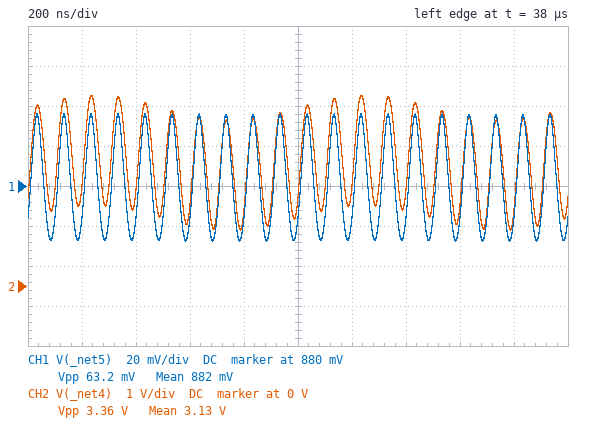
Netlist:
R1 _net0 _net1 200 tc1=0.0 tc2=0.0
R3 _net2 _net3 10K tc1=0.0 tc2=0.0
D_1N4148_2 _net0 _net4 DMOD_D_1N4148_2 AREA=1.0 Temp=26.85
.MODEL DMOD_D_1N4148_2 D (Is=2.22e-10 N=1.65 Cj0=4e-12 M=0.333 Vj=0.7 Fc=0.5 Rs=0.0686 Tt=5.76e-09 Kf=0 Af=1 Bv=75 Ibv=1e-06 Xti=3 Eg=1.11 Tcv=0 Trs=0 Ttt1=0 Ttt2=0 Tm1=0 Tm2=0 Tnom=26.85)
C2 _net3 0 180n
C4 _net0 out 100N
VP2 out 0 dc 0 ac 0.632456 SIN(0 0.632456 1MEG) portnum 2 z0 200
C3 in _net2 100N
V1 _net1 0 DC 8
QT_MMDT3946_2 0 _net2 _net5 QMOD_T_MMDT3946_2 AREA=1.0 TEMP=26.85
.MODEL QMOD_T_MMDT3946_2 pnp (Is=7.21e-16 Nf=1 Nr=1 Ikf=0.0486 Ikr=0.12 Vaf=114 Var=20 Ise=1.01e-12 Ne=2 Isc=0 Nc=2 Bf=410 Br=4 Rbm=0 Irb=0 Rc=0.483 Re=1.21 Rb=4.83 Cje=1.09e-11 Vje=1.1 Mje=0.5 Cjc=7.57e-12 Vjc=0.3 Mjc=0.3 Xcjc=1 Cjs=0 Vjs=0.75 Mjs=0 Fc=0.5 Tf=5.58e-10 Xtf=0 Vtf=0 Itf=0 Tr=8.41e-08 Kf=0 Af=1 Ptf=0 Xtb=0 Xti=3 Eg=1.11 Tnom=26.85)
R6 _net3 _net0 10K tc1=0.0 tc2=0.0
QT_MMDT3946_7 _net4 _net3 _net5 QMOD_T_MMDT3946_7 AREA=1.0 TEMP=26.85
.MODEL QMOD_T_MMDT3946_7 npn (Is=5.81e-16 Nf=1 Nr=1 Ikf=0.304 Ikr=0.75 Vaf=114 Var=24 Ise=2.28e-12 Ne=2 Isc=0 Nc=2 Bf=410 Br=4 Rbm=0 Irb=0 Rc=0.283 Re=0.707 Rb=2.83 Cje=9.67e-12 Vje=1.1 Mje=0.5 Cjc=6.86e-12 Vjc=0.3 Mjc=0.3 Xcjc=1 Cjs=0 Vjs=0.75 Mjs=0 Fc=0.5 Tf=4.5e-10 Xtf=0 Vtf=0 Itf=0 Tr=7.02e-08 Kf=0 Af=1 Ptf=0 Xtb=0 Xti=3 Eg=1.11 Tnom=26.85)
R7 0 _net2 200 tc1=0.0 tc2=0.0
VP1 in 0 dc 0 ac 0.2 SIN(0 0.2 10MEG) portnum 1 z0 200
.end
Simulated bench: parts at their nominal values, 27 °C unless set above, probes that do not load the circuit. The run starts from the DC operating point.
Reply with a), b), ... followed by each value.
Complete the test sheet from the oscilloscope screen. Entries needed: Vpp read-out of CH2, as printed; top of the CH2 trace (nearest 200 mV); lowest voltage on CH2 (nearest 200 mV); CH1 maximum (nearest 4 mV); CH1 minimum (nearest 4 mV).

a) 3.36 V
b) 4.8 V
c) 1.4 V
d) 916 mV
e) 852 mV
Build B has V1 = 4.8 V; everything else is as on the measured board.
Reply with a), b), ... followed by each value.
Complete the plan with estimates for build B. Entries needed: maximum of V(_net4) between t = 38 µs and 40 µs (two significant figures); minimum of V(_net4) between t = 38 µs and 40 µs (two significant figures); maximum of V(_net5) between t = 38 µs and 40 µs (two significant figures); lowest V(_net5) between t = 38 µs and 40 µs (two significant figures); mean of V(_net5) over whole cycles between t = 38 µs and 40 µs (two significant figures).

a) 3.5 V
b) 1.2 V
c) 860 mV
d) 780 mV
e) 820 mV
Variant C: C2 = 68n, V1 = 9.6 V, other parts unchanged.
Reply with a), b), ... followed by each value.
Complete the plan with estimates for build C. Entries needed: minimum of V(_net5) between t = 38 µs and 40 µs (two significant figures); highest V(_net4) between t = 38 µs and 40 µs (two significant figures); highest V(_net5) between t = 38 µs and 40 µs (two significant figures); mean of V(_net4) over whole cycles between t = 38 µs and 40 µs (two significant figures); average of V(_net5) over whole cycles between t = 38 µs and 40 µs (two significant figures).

a) 880 mV
b) 5.3 V
c) 940 mV
d) 3.5 V
e) 910 mV
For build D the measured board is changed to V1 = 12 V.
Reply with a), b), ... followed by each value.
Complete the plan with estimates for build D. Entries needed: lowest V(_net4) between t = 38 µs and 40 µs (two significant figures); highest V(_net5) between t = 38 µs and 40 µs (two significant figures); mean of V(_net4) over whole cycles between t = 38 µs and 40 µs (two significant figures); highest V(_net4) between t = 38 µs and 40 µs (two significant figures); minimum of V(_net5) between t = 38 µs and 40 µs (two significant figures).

a) 1.9 V
b) 970 mV
c) 3.9 V
d) 5.8 V
e) 920 mV
